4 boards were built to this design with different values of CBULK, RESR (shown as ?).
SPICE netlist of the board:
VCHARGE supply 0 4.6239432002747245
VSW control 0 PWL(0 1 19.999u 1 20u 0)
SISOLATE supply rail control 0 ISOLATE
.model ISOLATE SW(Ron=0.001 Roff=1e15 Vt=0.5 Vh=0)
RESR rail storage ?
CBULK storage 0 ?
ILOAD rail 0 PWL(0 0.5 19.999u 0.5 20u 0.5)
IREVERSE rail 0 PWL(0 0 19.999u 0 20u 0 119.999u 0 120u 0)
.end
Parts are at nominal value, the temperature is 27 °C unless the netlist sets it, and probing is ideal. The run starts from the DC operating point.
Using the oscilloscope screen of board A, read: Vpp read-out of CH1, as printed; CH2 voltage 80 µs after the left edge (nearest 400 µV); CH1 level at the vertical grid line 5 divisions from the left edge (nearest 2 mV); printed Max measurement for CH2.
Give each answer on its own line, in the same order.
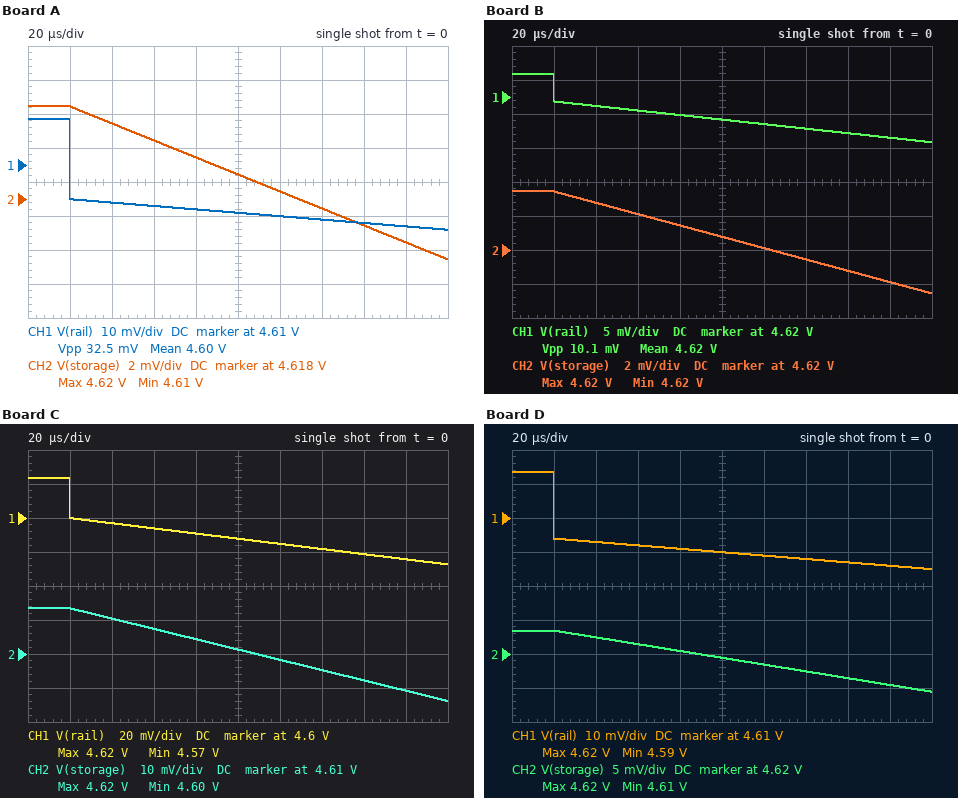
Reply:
32.5 mV
4.6204 V
4.596 V
4.62 V
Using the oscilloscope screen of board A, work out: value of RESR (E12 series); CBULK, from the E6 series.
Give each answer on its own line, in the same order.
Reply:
0.047 Ω
10 mF
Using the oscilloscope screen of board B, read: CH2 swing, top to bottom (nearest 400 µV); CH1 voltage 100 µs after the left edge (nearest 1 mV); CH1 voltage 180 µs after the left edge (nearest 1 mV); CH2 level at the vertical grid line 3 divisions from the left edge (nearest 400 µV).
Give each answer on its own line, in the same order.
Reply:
6.0 mV
4.617 V
4.614 V
4.6220 V
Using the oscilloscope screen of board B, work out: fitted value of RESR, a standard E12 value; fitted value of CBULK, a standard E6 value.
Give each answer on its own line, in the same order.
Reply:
8.2 mΩ
15 mF
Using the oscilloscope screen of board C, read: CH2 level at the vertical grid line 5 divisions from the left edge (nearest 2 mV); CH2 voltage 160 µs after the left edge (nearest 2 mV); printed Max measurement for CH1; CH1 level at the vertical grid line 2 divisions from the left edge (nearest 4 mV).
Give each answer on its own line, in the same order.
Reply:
4.612 V
4.602 V
4.62 V
4.596 V
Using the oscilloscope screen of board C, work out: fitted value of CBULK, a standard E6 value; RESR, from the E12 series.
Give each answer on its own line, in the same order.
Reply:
3.3 mF
0.047 Ω
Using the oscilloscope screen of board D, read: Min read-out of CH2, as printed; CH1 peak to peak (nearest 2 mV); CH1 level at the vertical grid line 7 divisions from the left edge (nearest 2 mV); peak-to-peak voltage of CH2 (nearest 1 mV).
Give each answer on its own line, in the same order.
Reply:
4.61 V
28 mV
4.598 V
9 mV
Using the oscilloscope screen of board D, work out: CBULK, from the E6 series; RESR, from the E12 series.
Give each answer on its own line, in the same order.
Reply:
10 mF
0.039 Ω
